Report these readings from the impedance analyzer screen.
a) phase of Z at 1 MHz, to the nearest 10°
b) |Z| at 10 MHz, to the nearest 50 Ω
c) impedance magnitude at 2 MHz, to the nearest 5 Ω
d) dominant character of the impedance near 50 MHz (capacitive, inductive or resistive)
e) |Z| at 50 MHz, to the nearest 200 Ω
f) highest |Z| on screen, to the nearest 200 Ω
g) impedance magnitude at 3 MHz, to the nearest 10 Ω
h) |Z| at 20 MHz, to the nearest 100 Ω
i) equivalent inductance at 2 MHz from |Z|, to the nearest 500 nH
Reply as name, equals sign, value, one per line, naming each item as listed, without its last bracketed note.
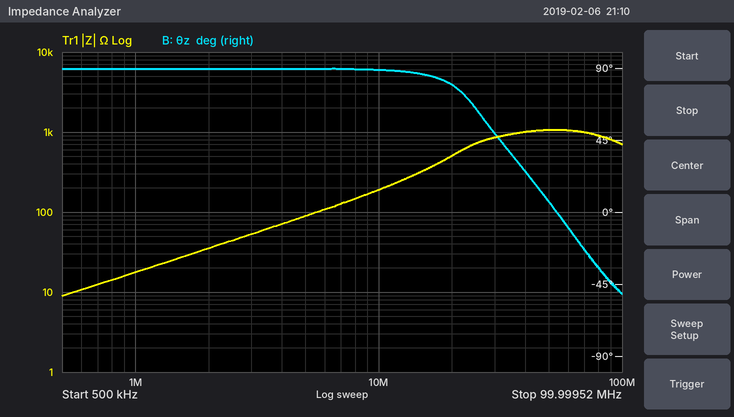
phase of Z at 1 MHz, to the nearest 10° = 90°
|Z| at 10 MHz, to the nearest 50 Ω = 200 Ω
impedance magnitude at 2 MHz, to the nearest 5 Ω = 35 Ω
dominant character of the impedance near 50 MHz = resistive
|Z| at 50 MHz, to the nearest 200 Ω = 1.0 kΩ
highest |Z| on screen, to the nearest 200 Ω = 1.0 kΩ
impedance magnitude at 3 MHz, to the nearest 10 Ω = 50 Ω
|Z| at 20 MHz, to the nearest 100 Ω = 500 Ω
equivalent inductance at 2 MHz from |Z|, to the nearest 500 nH = 3.0 µH
